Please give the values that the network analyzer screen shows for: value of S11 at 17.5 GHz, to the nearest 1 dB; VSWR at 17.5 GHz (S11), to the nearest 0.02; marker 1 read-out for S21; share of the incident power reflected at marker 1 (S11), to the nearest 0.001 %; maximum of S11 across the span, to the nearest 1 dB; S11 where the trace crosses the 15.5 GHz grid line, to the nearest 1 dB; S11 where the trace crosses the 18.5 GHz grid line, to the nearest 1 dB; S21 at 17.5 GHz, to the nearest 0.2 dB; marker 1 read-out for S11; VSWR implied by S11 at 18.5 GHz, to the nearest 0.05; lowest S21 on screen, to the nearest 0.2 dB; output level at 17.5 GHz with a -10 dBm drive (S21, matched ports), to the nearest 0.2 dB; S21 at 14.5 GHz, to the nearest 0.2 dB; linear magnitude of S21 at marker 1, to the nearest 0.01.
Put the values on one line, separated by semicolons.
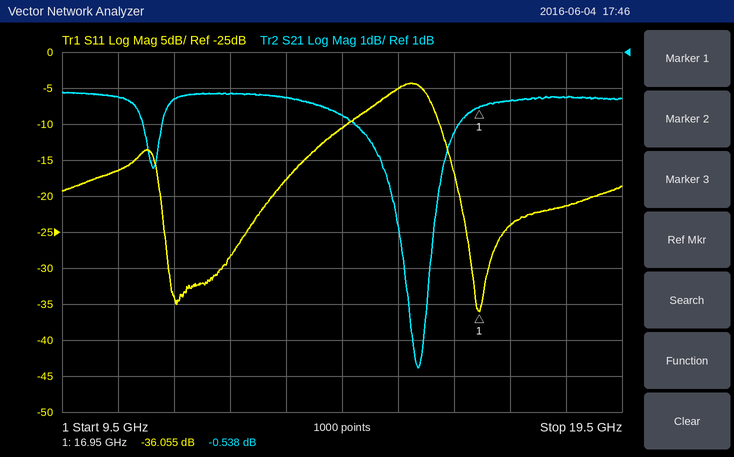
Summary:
-24 dB; 1.14; -0.538 dB; 0.025 %; -4 dB; -5 dB; -21 dB; -0.4 dB; -36.055 dB; 1.20; -7.8 dB; -10.4 dBm; -0.8 dB; 0.94
